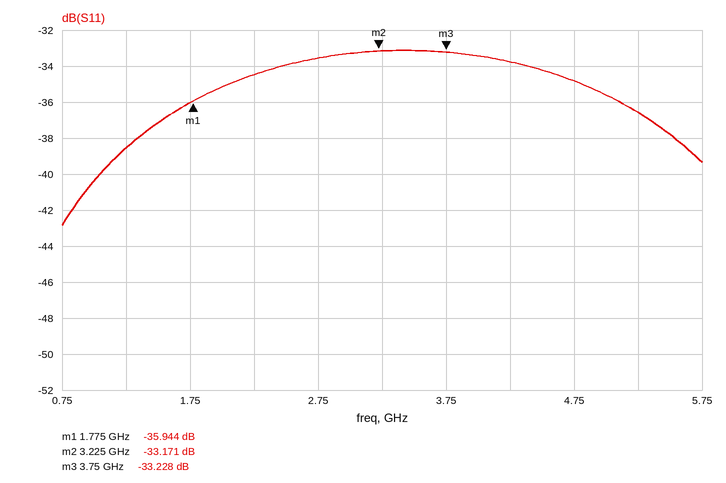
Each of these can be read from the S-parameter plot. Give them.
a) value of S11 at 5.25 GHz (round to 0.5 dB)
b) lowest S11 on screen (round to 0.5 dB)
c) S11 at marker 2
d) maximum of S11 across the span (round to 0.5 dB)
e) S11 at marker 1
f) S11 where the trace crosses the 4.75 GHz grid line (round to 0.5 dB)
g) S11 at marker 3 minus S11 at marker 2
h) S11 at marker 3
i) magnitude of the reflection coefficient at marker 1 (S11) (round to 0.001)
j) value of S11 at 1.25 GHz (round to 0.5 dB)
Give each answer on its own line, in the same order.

-36.5 dB
-43.0 dB
-33.171 dB
-33.0 dB
-35.944 dB
-35.0 dB
-0.057 dB
-33.228 dB
0.016
-38.5 dB
